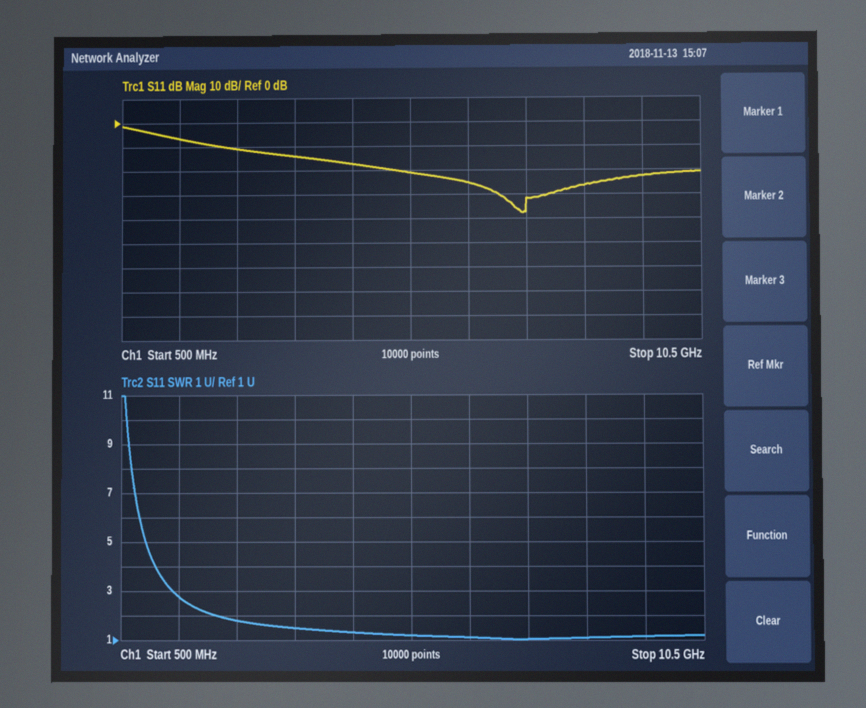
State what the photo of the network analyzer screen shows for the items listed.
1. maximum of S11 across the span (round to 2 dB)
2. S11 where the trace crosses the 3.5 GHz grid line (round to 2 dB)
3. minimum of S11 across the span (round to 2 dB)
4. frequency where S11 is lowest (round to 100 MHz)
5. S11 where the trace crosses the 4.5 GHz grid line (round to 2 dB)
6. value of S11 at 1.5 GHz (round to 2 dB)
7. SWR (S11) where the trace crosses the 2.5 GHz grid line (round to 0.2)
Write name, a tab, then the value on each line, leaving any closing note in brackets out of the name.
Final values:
maximum of S11 across the span	-2 dB
S11 where the trace crosses the 3.5 GHz grid line	-14 dB
minimum of S11 across the span	-38 dB
frequency where S11 is lowest	7.4 GHz
S11 where the trace crosses the 4.5 GHz grid line	-18 dB
value of S11 at 1.5 GHz	-6 dB
SWR (S11) where the trace crosses the 2.5 GHz grid line	1.8
